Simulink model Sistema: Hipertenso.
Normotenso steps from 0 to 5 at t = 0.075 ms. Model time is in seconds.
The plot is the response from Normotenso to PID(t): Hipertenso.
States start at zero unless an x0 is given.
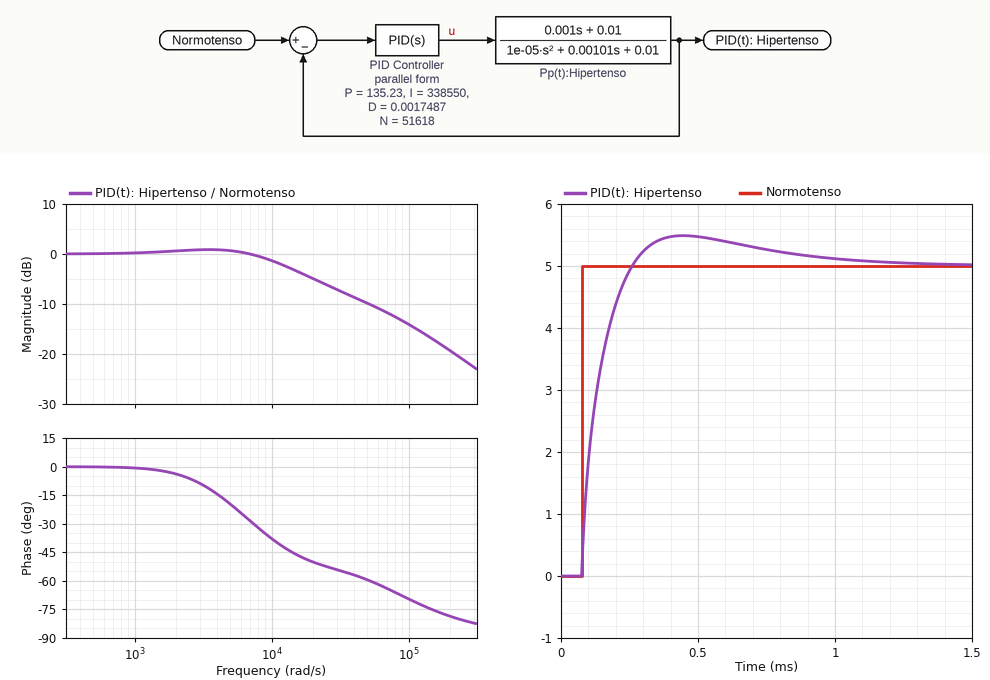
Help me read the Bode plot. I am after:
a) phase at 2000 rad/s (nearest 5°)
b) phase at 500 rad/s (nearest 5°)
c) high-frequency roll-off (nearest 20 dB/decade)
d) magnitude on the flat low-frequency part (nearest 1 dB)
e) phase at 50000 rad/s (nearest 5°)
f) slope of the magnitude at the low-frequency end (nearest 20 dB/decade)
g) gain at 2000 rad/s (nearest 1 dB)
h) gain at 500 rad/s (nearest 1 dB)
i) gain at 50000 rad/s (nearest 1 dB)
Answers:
-5°
0°
-20 dB/decade
0 dB
-60°
0 dB/decade
1 dB
0 dB
-10 dB
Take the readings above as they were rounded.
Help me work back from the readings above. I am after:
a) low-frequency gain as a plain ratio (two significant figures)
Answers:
1.0
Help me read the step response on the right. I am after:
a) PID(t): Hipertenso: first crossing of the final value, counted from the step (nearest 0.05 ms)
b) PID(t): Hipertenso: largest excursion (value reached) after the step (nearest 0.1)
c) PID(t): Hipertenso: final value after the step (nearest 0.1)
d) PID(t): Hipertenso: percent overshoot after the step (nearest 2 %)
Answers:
0.20 ms
5.5
5.0
10 %
